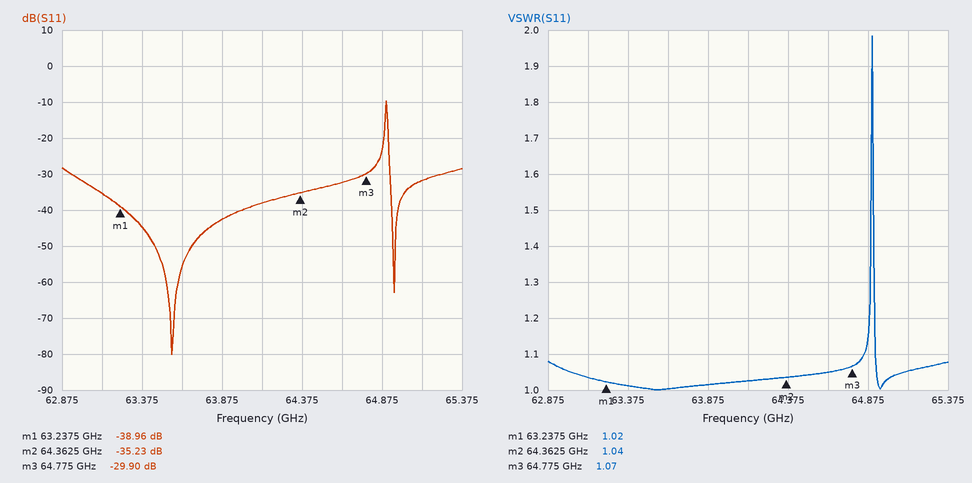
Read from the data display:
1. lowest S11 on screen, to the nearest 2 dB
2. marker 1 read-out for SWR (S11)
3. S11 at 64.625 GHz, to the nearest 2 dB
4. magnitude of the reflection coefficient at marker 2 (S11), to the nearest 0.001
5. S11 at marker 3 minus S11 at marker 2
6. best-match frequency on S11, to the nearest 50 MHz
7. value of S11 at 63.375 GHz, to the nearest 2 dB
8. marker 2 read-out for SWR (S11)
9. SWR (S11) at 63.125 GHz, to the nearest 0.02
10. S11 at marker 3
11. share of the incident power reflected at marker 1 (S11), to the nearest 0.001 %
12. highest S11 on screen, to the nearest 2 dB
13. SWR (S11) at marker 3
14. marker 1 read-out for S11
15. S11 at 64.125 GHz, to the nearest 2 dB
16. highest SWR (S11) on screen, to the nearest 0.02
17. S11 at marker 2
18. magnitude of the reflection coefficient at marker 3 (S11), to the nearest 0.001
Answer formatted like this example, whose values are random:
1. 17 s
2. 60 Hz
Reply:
1. -80 dB
2. 1.02
3. -32 dB
4. 0.017
5. 5.33 dB
6. 63.55 GHz
7. -44 dB
8. 1.04
9. 1.04
10. -29.90 dB
11. 0.013 %
12. -10 dB
13. 1.07
14. -38.96 dB
15. -38 dB
16. 1.98
17. -35.23 dB
18. 0.032
